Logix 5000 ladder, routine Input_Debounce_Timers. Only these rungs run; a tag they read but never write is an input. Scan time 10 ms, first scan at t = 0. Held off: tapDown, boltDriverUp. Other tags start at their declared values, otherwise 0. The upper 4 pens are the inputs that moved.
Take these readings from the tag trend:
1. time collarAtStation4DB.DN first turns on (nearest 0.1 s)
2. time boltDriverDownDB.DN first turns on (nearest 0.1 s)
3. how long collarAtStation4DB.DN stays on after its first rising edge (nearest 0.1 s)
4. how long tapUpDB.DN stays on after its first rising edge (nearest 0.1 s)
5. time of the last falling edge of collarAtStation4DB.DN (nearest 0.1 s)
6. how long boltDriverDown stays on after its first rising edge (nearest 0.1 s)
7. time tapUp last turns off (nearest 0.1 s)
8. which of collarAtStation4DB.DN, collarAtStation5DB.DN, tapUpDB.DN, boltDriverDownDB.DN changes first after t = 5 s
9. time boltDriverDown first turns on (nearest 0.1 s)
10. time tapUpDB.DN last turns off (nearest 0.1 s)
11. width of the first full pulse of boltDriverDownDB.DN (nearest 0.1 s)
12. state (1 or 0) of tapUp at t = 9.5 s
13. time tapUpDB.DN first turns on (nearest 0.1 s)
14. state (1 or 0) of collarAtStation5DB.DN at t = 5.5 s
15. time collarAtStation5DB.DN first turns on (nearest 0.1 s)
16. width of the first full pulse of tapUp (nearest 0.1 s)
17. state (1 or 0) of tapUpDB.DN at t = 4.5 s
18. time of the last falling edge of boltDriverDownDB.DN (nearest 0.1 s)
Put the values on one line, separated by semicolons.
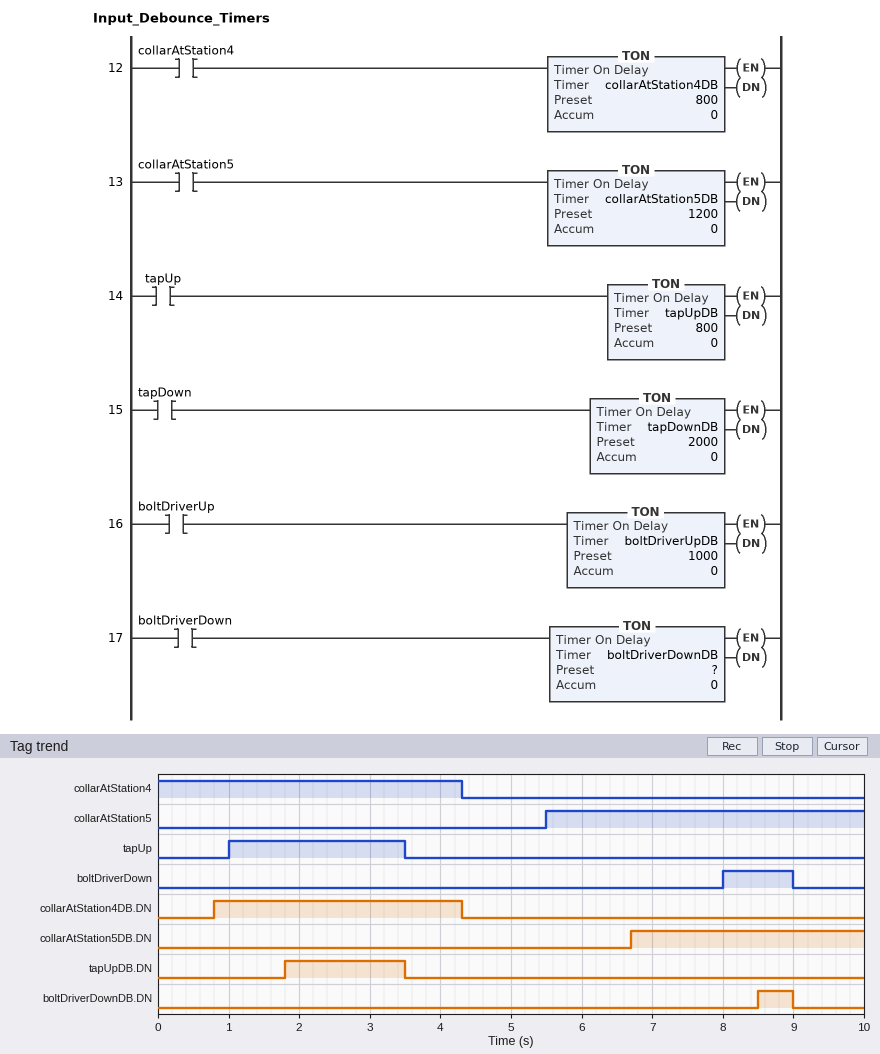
0.8 s; 8.5 s; 3.5 s; 1.7 s; 4.3 s; 1.0 s; 3.5 s; collarAtStation5DB.DN; 8.0 s; 3.5 s; 0.5 s; 0; 1.8 s; 0; 6.7 s; 2.5 s; 0; 9.0 s
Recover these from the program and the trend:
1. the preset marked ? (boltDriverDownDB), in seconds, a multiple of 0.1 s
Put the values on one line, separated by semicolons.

0.5 s
